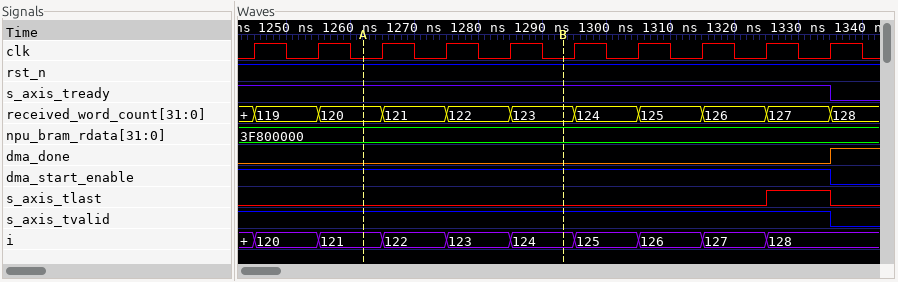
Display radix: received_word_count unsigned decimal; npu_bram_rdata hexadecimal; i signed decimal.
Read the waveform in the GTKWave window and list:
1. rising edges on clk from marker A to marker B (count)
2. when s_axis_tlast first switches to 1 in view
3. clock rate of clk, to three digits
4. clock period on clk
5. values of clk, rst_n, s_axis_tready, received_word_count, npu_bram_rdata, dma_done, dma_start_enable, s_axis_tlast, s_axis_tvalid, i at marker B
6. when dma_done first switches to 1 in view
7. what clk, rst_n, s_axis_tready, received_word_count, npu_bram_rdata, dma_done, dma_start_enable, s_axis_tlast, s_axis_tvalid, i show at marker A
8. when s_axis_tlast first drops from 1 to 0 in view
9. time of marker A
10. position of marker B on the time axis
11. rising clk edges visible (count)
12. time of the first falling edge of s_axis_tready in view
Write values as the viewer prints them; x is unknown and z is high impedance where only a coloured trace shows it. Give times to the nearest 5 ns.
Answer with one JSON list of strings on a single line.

["3", "1325 ns", "100 MHz", "10 ns", "clk=0, rst_n=1, s_axis_tready=1, received_word_count=123, npu_bram_rdata=3F800000, dma_done=0, dma_start_enable=1, s_axis_tlast=0, s_axis_tvalid=1, i=124", "1335 ns", "clk=0, rst_n=1, s_axis_tready=1, received_word_count=120, npu_bram_rdata=3F800000, dma_done=0, dma_start_enable=1, s_axis_tlast=0, s_axis_tvalid=1, i=121", "1335 ns", "1260 ns", "1295 ns", "10", "1335 ns"]
